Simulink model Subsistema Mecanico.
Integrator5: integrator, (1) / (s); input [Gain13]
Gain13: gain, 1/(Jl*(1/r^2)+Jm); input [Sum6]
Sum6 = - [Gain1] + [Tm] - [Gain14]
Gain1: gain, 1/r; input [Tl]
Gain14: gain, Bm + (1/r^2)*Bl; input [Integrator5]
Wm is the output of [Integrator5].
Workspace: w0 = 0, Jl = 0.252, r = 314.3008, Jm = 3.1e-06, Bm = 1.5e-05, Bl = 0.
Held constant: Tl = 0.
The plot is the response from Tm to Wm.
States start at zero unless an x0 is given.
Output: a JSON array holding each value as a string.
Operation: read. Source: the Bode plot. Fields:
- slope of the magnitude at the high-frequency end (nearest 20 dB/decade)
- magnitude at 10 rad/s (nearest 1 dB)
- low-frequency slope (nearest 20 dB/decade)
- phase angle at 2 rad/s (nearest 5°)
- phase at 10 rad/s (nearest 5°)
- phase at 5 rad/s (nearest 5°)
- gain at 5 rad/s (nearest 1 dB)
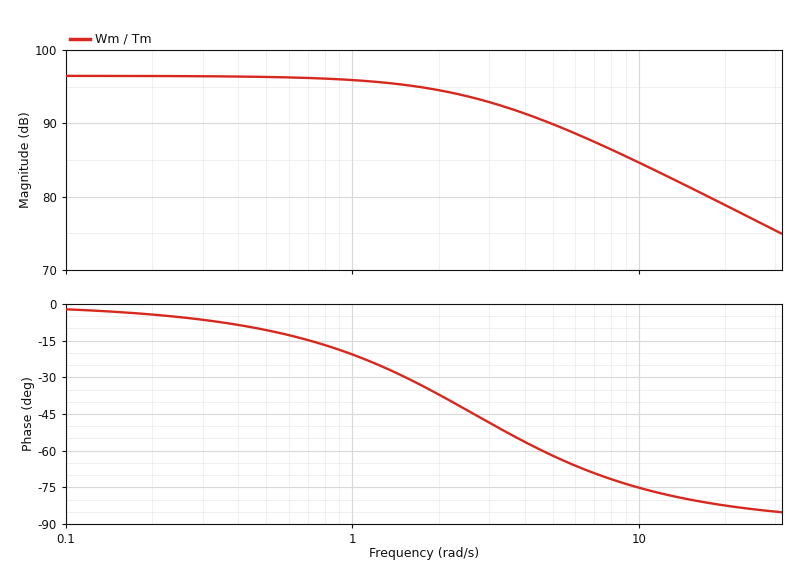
["-20 dB/decade", "85 dB", "0 dB/decade", "-35°", "-75°", "-60°", "90 dB"]
